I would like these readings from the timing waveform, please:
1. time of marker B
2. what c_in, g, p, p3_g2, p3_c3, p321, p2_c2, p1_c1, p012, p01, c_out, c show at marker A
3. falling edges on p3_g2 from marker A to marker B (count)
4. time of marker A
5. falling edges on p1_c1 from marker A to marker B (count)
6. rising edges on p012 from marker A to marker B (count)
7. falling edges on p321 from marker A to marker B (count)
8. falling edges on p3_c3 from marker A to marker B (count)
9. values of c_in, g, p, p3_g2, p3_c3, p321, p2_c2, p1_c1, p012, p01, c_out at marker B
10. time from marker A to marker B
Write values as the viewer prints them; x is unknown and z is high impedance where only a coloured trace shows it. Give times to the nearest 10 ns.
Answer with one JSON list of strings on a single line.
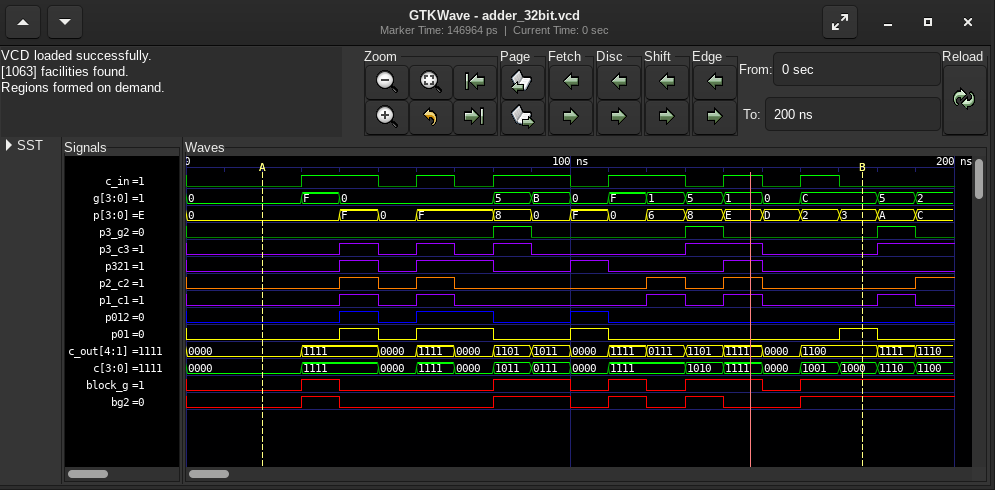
["180 ns", "c_in=0, g=0, p=0, p3_g2=0, p3_c3=0, p321=0, p2_c2=0, p1_c1=0, p012=0, p01=0, c_out=0000, c=0000", "2", "20 ns", "4", "3", "4", "4", "c_in=0, g=C, p=3, p3_g2=0, p3_c3=0, p321=0, p2_c2=0, p1_c1=0, p012=0, p01=1, c_out=1100", "160 ns"]
